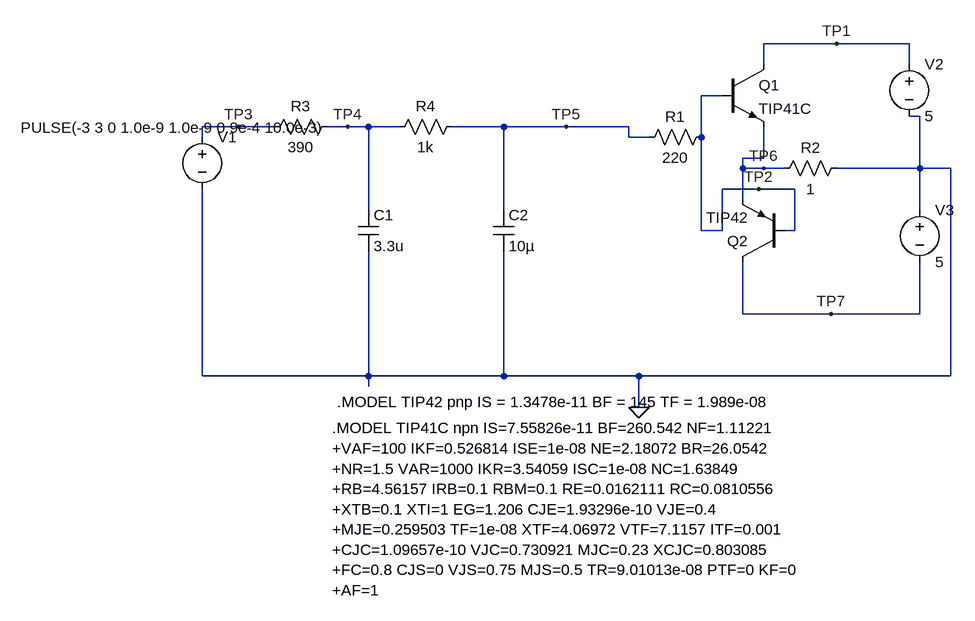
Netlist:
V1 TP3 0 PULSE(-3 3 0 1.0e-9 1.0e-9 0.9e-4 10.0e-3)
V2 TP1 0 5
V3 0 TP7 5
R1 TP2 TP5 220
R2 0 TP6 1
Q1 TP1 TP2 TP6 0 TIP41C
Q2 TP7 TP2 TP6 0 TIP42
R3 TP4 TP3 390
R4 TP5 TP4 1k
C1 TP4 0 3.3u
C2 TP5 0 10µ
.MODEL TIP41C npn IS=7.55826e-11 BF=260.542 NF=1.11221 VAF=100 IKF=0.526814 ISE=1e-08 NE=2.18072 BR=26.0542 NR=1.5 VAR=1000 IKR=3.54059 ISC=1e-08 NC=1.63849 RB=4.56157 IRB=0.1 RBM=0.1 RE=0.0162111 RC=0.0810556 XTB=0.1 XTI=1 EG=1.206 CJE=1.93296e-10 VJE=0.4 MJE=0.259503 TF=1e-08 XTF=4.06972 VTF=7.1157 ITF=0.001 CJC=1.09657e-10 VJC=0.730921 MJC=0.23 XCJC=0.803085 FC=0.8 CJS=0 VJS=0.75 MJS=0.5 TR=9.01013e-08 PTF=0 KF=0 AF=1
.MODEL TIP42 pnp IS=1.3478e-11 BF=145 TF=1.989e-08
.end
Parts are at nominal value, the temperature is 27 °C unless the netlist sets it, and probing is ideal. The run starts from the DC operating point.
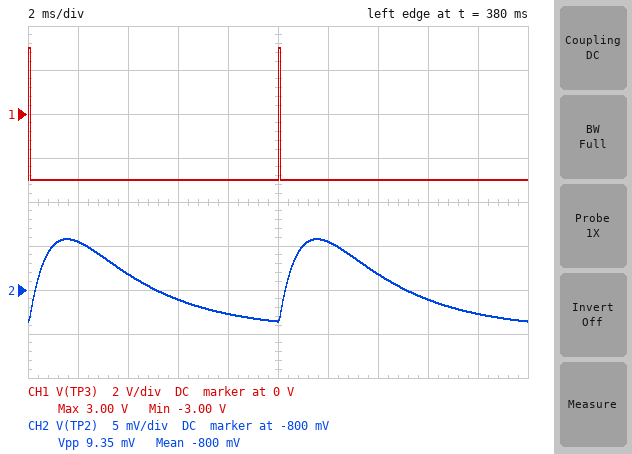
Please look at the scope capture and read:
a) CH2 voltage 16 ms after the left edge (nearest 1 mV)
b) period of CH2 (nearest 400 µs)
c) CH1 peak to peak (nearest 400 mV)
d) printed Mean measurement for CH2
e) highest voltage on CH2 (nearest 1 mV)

-801 mV
10.0 ms
6.0 V
-800 mV
-794 mV
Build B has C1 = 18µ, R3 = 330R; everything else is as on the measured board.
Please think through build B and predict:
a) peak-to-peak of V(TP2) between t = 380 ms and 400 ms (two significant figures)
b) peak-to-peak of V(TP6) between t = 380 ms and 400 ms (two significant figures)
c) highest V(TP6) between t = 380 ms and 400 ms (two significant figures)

3.7 mV
3.3 mV
-200 mV
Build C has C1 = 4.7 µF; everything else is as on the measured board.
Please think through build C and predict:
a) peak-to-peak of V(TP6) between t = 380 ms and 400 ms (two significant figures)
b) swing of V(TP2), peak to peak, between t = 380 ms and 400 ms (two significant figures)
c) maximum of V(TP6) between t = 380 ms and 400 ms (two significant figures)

7.1 mV
8.1 mV
-190 mV
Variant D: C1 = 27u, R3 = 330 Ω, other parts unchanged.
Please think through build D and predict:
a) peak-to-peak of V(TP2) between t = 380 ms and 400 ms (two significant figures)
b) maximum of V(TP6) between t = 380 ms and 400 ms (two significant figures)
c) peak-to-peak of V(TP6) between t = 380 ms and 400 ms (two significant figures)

2.6 mV
-200 mV
2.3 mV
